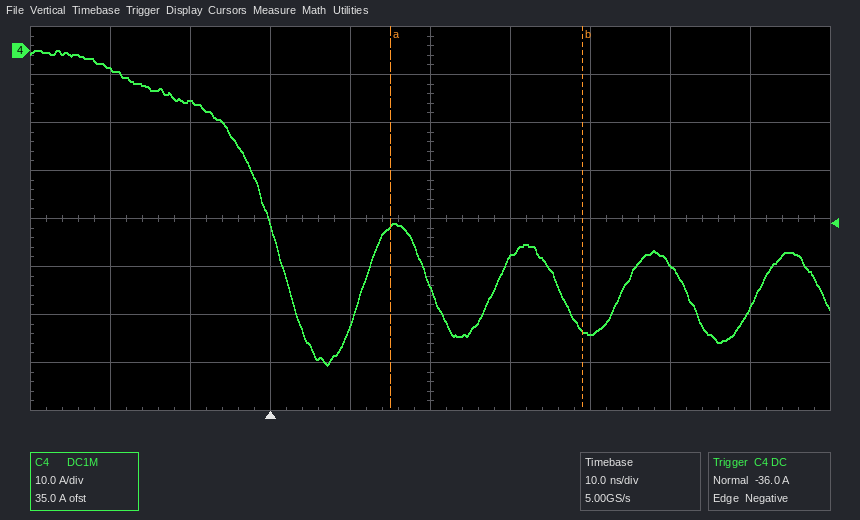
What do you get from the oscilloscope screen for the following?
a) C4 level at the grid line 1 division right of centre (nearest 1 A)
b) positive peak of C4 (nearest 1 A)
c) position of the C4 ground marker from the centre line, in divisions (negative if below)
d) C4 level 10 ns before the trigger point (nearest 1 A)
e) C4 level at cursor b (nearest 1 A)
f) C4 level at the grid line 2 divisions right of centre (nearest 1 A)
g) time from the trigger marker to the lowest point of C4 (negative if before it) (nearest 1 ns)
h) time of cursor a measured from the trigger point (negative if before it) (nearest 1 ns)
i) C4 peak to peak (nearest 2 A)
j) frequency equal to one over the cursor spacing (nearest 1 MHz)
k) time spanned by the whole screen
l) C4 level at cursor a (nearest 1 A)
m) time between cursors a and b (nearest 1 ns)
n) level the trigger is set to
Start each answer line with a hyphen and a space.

- -43 A
- 0 A
- +3.5 div
- -11 A
- -58 A
- -59 A
- +7 ns
- +15 ns
- 66 A
- 42 MHz
- 100 ns
- -37 A
- 24 ns
- -36.0 A
